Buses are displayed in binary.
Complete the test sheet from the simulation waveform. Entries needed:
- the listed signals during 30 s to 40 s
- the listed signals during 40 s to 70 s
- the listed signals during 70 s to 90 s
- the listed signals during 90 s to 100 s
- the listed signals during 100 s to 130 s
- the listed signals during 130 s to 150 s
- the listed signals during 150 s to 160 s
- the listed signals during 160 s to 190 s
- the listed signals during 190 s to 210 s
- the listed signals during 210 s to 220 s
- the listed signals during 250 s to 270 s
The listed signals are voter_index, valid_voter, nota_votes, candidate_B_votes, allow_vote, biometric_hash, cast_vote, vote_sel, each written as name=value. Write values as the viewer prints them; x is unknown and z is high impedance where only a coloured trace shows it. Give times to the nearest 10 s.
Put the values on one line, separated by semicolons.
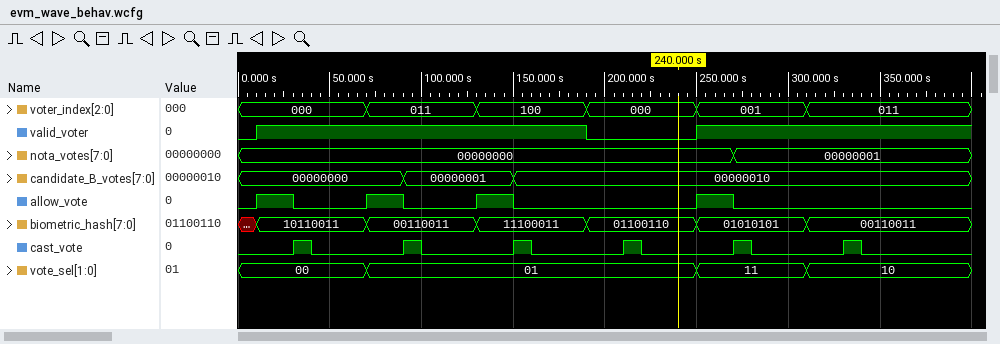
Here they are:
voter_index=000, valid_voter=1, nota_votes=00000000, candidate_B_votes=00000000, allow_vote=0, biometric_hash=10110011, cast_vote=1, vote_sel=00; voter_index=000, valid_voter=1, nota_votes=00000000, candidate_B_votes=00000000, allow_vote=0, biometric_hash=10110011, cast_vote=0, vote_sel=00; voter_index=011, valid_voter=1, nota_votes=00000000, candidate_B_votes=00000000, allow_vote=1, biometric_hash=00110011, cast_vote=0, vote_sel=01; voter_index=011, valid_voter=1, nota_votes=00000000, candidate_B_votes=00000001, allow_vote=0, biometric_hash=00110011, cast_vote=1, vote_sel=01; voter_index=011, valid_voter=1, nota_votes=00000000, candidate_B_votes=00000001, allow_vote=0, biometric_hash=00110011, cast_vote=0, vote_sel=01; voter_index=100, valid_voter=1, nota_votes=00000000, candidate_B_votes=00000001, allow_vote=1, biometric_hash=11100011, cast_vote=0, vote_sel=01; voter_index=100, valid_voter=1, nota_votes=00000000, candidate_B_votes=00000010, allow_vote=0, biometric_hash=11100011, cast_vote=1, vote_sel=01; voter_index=100, valid_voter=1, nota_votes=00000000, candidate_B_votes=00000010, allow_vote=0, biometric_hash=11100011, cast_vote=0, vote_sel=01; voter_index=000, valid_voter=0, nota_votes=00000000, candidate_B_votes=00000010, allow_vote=0, biometric_hash=01100110, cast_vote=0, vote_sel=01; voter_index=000, valid_voter=0, nota_votes=00000000, candidate_B_votes=00000010, allow_vote=0, biometric_hash=01100110, cast_vote=1, vote_sel=01; voter_index=001, valid_voter=1, nota_votes=00000000, candidate_B_votes=00000010, allow_vote=1, biometric_hash=01010101, cast_vote=0, vote_sel=11
